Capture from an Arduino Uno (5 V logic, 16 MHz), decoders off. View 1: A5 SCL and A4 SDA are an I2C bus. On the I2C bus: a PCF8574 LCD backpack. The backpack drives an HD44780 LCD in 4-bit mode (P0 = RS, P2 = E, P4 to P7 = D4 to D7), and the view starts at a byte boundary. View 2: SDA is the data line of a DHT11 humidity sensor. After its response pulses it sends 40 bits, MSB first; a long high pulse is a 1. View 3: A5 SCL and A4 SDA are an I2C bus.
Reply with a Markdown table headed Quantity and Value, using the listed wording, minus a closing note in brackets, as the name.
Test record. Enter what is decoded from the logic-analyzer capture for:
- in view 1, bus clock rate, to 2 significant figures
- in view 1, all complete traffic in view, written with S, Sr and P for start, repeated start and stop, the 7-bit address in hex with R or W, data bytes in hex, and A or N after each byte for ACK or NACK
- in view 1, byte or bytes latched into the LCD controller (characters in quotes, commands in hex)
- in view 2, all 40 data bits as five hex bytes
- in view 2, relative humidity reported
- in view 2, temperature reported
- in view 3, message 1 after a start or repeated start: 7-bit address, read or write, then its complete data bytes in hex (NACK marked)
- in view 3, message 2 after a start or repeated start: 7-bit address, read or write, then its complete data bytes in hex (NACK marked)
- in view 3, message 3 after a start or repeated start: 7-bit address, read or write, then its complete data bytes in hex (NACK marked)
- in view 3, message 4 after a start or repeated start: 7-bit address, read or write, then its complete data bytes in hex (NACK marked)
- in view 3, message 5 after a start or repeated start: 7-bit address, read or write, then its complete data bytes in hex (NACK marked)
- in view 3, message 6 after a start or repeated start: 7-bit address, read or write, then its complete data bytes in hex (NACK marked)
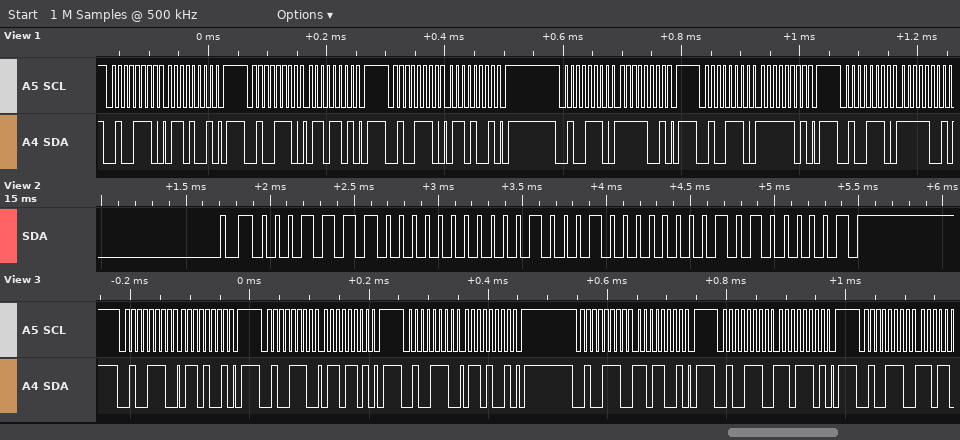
| Quantity | Value |
|---|---|
| in view 1, bus clock rate, to 2 significant figures | 100 kHz |
| in view 1, all complete traffic in view, written with S, Sr and P for start, repeated start and stop, the 7-bit address in hex with R or W, data bytes in hex, and A or N after each byte for ACK or NACK | S 27W A 69 A P S 27W A 6D A P S 27W A 69 A P S 27W A F9 A P S 27W A FD A P S 27W A F9 A |
| in view 1, byte or bytes latched into the LCD controller | 'o' |
| in view 2, all 40 data bits as five hex bytes | 1E 00 22 01 41 |
| in view 2, relative humidity reported | 30 % |
| in view 2, temperature reported | 34.1 °C |
| in view 3, message 1 after a start or repeated start: 7-bit address, read or write, then its complete data bytes in hex | 0x27 write: 69 |
| in view 3, message 2 after a start or repeated start: 7-bit address, read or write, then its complete data bytes in hex | 0x27 write: 6D |
| in view 3, message 3 after a start or repeated start: 7-bit address, read or write, then its complete data bytes in hex | 0x27 write: 69 |
| in view 3, message 4 after a start or repeated start: 7-bit address, read or write, then its complete data bytes in hex | 0x27 write: D9 |
| in view 3, message 5 after a start or repeated start: 7-bit address, read or write, then its complete data bytes in hex | 0x27 write: DD |
| in view 3, message 6 after a start or repeated start: 7-bit address, read or write, then its complete data bytes in hex | 0x27 write |
